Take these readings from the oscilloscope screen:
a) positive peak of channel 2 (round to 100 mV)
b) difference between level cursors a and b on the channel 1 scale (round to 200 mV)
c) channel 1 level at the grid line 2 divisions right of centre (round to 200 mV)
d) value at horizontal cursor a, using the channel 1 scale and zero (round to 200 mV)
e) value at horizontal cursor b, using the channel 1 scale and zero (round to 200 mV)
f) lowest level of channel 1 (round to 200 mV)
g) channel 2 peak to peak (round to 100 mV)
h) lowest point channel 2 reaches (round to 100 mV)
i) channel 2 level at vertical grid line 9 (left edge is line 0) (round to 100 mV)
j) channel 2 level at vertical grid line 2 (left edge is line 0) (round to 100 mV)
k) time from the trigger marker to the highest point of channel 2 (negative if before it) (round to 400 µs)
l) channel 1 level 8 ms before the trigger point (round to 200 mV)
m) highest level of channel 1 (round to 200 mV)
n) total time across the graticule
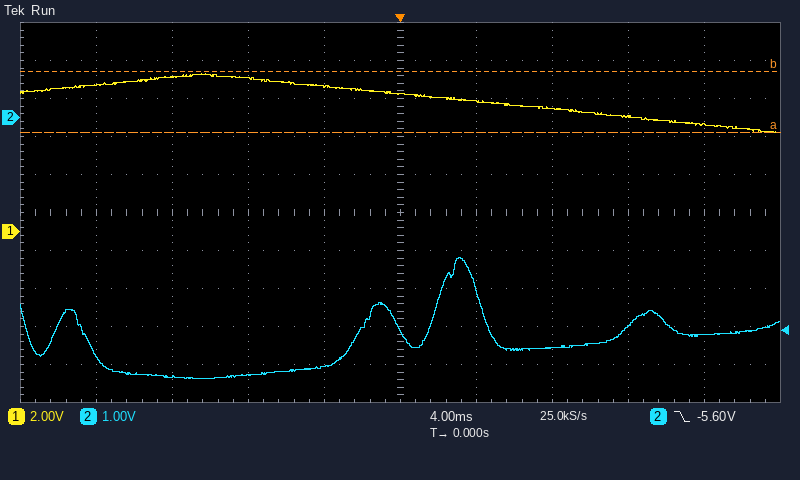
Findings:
-3.7 V
3.2 V
6.4 V
5.2 V
8.4 V
5.2 V
3.2 V
-6.9 V
-5.7 V
-6.8 V
+3.2 ms
8.0 V
8.4 V
40 ms
